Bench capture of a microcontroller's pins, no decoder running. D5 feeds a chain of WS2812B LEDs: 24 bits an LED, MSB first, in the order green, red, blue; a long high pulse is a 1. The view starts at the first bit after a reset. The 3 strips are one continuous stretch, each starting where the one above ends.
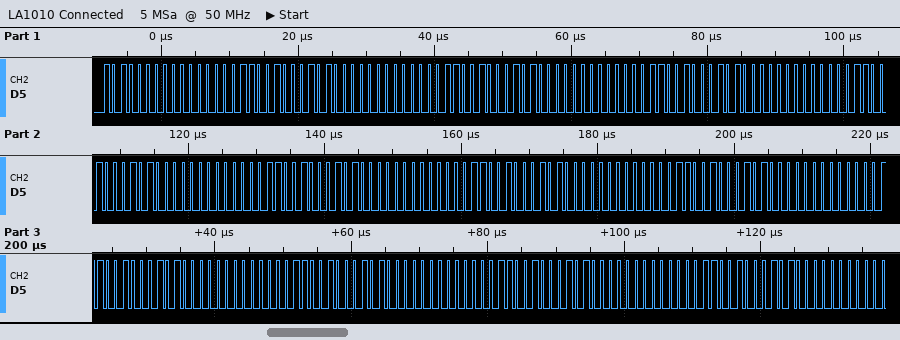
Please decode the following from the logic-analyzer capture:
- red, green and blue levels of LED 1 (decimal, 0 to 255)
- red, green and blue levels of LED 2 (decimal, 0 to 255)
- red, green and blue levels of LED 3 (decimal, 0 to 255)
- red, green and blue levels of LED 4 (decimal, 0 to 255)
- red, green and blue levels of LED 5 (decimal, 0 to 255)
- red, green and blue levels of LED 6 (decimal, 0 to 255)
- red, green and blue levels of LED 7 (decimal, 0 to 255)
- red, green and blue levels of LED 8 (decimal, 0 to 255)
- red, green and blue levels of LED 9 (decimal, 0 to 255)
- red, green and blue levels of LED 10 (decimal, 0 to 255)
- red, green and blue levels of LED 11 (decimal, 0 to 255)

0, 160, 200
0, 160, 200
0, 160, 200
0, 160, 200
0, 160, 200
0, 160, 200
0, 160, 200
0, 160, 200
0, 160, 200
0, 160, 200
0, 160, 200
